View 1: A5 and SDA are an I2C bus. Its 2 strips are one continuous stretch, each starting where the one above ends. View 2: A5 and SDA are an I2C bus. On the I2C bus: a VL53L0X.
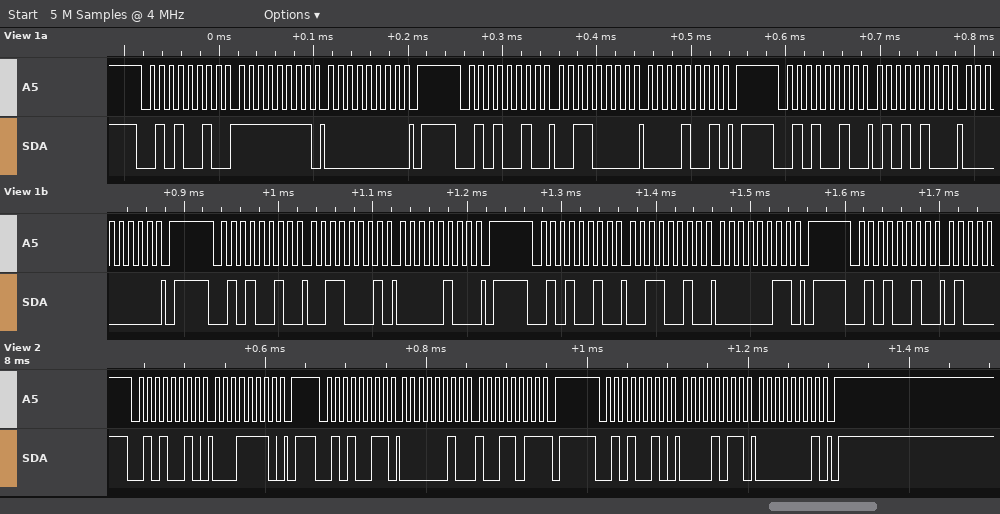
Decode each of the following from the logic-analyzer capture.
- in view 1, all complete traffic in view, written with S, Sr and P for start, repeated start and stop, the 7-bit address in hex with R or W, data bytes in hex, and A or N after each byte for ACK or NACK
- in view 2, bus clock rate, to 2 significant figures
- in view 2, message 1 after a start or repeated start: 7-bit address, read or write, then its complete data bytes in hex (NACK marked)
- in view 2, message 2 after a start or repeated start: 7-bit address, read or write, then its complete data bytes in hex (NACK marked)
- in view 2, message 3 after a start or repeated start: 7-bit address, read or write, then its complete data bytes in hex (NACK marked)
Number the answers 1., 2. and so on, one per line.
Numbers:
1. S 29W A FF A 00 A P S 29W A 30 A 09 A P S 29W A 54 A 00 A P S 29W A 31 A 04 A P S 29W A 32 A 03 A P S 29W A
2. 100 kHz
3. 0x29 write: 1E
4. 0x29 read: 02 9B NACK
5. 0x29 write: 0B 01
